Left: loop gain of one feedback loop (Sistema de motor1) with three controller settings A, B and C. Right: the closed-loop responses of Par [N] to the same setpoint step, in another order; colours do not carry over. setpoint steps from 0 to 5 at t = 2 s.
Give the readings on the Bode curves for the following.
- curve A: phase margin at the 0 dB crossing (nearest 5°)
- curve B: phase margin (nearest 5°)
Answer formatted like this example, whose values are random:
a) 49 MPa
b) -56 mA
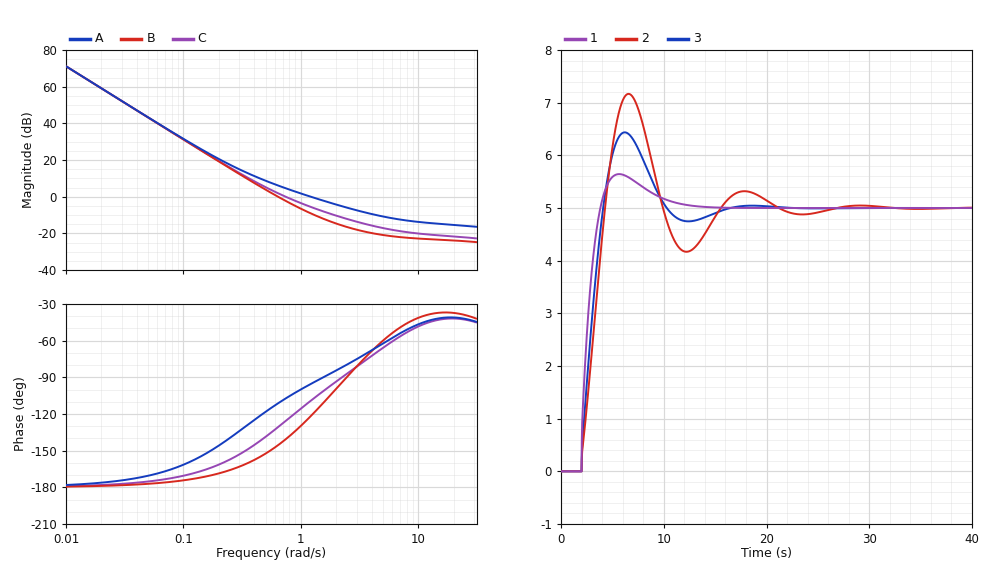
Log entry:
a) 85°
b) 35°
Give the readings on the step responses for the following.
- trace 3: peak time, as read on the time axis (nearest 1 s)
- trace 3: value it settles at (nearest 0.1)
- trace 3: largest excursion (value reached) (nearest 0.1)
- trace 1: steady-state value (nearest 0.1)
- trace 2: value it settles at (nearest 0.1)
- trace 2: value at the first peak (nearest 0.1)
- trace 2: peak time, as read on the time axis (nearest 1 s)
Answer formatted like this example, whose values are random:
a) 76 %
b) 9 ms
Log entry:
a) 6 s
b) 5.0
c) 6.4
d) 5.0
e) 5.0
f) 7.2
g) 7 s
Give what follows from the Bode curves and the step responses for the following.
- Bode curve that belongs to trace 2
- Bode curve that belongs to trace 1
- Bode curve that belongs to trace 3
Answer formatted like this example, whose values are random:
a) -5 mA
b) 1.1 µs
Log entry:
a) B
b) A
c) C
